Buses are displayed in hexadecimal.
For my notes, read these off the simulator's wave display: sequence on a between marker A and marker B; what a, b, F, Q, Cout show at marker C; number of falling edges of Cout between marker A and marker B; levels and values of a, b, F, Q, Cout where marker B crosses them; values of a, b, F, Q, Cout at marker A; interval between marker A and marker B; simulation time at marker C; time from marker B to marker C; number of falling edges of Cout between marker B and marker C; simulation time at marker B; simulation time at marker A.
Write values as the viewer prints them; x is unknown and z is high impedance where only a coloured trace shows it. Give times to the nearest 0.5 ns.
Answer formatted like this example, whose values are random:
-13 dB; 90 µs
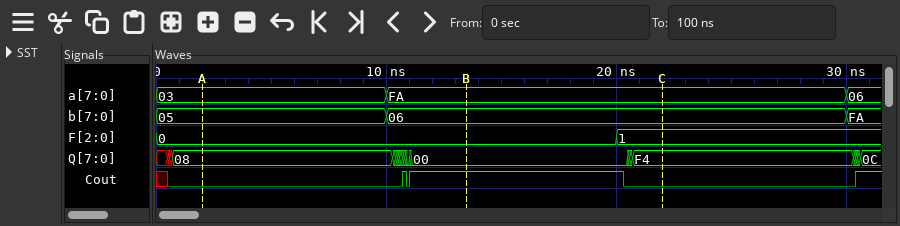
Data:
03, FA; a=FA, b=06, F=1, Q=F4, Cout=0; 1; a=FA, b=06, F=0, Q=00, Cout=1; a=03, b=05, F=0, Q=08, Cout=0; 11.5 ns; 22 ns; 8.5 ns; 1; 13.5 ns; 2 ns
